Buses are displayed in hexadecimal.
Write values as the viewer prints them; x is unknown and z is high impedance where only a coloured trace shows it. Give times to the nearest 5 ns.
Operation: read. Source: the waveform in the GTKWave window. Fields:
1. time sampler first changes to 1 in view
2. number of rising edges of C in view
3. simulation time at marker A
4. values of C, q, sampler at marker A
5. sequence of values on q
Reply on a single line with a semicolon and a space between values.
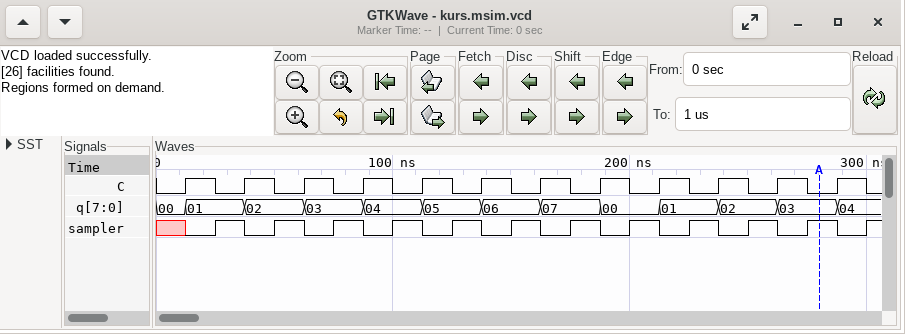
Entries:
25 ns; 12; 280 ns; C=0, q=03, sampler=1; 00, 01, 02, 03, 04, 05, 06, 07, 00, 01, 02, 03, 04
